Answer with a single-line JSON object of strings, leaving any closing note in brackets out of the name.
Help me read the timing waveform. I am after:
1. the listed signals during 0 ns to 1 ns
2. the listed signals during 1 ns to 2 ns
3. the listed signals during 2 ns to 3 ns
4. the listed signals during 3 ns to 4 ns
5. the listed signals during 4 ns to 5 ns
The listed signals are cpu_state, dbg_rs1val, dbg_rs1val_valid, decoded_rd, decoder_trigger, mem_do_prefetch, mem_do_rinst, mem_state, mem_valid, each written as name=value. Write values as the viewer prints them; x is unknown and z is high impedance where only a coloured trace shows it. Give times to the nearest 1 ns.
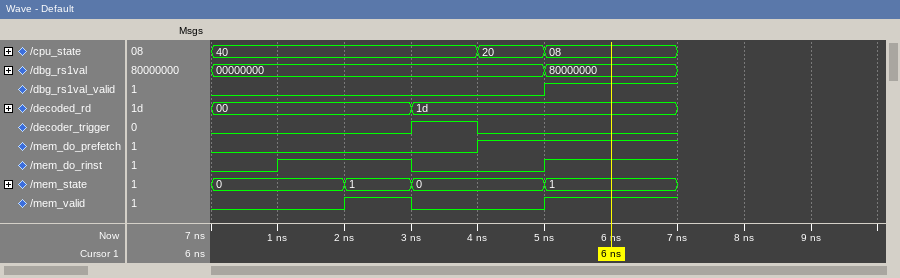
{"the listed signals during 0 ns to 1 ns": "cpu_state=40, dbg_rs1val=00000000, dbg_rs1val_valid=0, decoded_rd=00, decoder_trigger=0, mem_do_prefetch=0, mem_do_rinst=0, mem_state=0, mem_valid=0", "the listed signals during 1 ns to 2 ns": "cpu_state=40, dbg_rs1val=00000000, dbg_rs1val_valid=0, decoded_rd=00, decoder_trigger=0, mem_do_prefetch=0, mem_do_rinst=1, mem_state=0, mem_valid=0", "the listed signals during 2 ns to 3 ns": "cpu_state=40, dbg_rs1val=00000000, dbg_rs1val_valid=0, decoded_rd=00, decoder_trigger=0, mem_do_prefetch=0, mem_do_rinst=1, mem_state=1, mem_valid=1", "the listed signals during 3 ns to 4 ns": "cpu_state=40, dbg_rs1val=00000000, dbg_rs1val_valid=0, decoded_rd=1d, decoder_trigger=1, mem_do_prefetch=0, mem_do_rinst=0, mem_state=0, mem_valid=0", "the listed signals during 4 ns to 5 ns": "cpu_state=20, dbg_rs1val=00000000, dbg_rs1val_valid=0, decoded_rd=1d, decoder_trigger=0, mem_do_prefetch=1, mem_do_rinst=0, mem_state=0, mem_valid=0"}
